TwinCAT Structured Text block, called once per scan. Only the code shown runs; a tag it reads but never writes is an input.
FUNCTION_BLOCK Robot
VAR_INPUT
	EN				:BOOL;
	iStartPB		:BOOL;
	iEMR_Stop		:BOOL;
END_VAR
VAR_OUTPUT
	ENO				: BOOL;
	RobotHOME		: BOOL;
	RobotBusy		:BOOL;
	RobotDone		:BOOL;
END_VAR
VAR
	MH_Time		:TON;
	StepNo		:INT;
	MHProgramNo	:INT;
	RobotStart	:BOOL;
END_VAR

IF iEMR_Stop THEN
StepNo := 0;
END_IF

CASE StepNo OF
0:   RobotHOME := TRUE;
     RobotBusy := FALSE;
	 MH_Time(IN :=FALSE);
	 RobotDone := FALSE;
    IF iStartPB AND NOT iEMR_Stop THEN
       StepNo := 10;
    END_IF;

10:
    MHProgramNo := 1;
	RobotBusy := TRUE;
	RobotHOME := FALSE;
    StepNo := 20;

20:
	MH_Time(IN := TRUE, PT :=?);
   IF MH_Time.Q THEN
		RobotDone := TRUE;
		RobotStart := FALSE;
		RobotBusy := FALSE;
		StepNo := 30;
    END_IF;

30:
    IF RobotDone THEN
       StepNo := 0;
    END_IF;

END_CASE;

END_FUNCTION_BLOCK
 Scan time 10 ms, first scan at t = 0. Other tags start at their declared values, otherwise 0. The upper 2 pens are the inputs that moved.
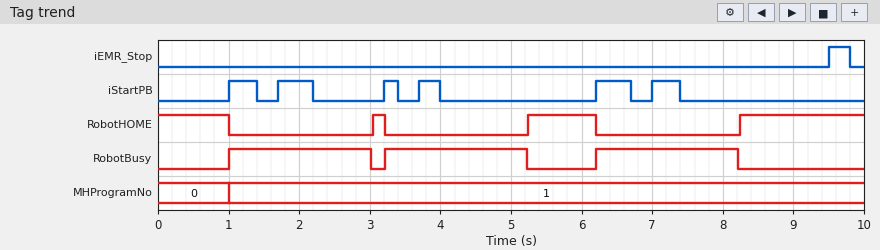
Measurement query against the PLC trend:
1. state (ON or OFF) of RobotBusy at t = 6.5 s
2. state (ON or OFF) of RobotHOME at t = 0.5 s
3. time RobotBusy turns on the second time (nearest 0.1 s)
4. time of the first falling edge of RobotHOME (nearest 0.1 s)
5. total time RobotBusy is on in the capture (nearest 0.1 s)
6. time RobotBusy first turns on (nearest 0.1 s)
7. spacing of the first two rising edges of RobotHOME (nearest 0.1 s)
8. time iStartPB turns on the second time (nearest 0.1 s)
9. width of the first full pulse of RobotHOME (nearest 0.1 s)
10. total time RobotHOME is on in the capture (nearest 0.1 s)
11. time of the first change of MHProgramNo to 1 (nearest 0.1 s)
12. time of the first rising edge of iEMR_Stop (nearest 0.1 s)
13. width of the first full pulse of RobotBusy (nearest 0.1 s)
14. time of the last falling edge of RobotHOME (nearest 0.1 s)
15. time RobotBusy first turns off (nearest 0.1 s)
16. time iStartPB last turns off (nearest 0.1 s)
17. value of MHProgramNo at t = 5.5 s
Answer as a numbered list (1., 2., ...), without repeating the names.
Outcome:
1. ON
2. ON
3. 3.2 s
4. 1.0 s
5. 6.0 s
6. 1.0 s
7. 2.2 s
8. 1.7 s
9. 0.2 s
10. 3.9 s
11. 1.0 s
12. 9.5 s
13. 2.0 s
14. 6.2 s
15. 3.0 s
16. 7.4 s
17. 1
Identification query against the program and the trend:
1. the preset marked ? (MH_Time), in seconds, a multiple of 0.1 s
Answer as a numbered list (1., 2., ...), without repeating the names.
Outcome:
1. 2.0 s
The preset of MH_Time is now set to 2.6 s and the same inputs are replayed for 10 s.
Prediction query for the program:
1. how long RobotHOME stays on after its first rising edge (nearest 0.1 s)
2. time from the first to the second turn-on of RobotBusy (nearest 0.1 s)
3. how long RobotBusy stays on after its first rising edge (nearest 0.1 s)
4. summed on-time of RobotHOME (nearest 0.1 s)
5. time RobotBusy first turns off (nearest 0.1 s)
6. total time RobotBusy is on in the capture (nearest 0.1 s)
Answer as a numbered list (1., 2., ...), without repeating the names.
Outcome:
1. 0.1 s
2. 2.7 s
3. 2.6 s
4. 2.1 s
5. 3.6 s
6. 7.8 s
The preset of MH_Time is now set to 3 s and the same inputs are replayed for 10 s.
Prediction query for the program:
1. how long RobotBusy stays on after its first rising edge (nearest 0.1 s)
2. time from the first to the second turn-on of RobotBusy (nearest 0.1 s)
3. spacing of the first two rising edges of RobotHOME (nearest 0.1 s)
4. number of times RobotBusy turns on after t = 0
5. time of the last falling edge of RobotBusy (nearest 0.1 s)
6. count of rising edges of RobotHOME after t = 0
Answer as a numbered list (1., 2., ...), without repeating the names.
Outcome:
1. 3.0 s
2. 5.2 s
3. 5.2 s
4. 2
5. 9.2 s
6. 2
